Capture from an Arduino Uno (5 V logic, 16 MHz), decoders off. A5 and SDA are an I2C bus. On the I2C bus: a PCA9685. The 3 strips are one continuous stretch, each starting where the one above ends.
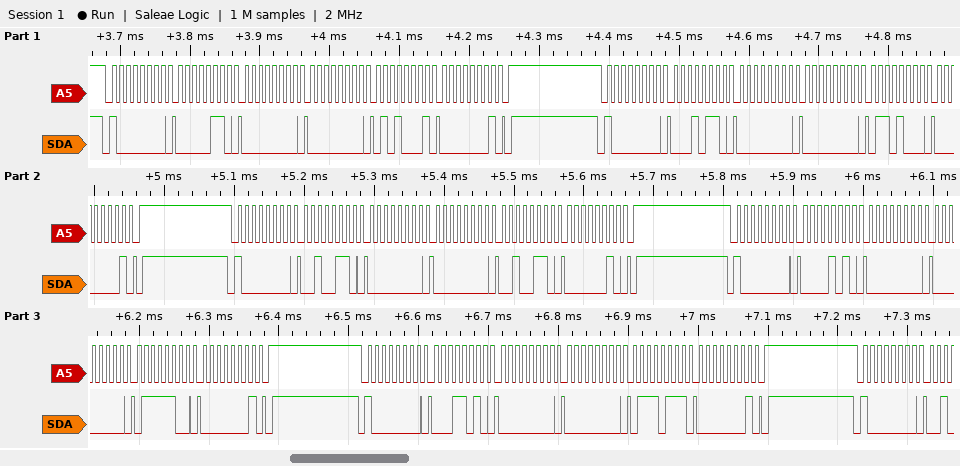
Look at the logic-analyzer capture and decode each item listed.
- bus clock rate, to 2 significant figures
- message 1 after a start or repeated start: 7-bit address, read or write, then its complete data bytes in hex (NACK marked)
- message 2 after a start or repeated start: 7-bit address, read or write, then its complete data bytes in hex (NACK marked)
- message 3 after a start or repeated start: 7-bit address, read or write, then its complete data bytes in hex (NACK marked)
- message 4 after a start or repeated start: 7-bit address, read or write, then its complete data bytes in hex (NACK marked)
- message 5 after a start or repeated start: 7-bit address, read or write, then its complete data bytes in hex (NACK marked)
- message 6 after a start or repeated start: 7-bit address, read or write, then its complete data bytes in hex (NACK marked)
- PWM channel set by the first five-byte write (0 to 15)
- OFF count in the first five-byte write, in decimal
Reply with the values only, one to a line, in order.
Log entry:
100 kHz
0x40 write: 06 00 00 51 01
0x40 write: 16 00 00 68 01
0x40 write: 26 00 00 26 02
0x40 write: 0A 00 00 7C 01
0x40 write: 1A 00 00 77 01
0x40 write
0
337
